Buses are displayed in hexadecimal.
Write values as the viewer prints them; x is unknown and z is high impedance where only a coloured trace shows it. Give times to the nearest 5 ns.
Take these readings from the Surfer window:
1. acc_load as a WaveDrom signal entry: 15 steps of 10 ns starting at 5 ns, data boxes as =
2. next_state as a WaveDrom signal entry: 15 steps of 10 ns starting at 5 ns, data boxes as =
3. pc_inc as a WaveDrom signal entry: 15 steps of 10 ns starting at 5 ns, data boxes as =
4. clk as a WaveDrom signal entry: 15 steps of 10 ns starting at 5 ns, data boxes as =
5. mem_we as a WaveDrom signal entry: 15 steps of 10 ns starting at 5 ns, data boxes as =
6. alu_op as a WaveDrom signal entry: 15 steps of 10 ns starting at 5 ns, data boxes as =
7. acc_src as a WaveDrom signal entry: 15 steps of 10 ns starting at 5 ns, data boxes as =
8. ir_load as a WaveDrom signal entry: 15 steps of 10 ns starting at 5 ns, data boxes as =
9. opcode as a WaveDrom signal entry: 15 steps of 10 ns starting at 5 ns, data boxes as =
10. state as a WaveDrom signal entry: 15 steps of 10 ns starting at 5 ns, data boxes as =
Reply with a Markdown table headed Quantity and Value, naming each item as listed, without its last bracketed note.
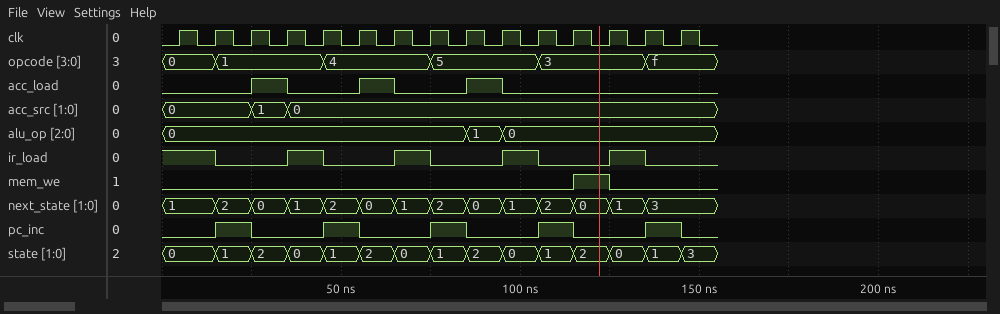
| Quantity | Value |
|---|---|
| acc_load as a WaveDrom signal entry: 15 steps of 10 ns starting at 5 ns, data boxes as = | {name: 'acc_load', wave: '0.10.10.10.....'} |
| next_state as a WaveDrom signal entry: 15 steps of 10 ns starting at 5 ns, data boxes as = | {name: 'next_state', wave: '==============.', data: '1 2 0 1 2 0 1 2 0 1 2 0 1 3'} |
| pc_inc as a WaveDrom signal entry: 15 steps of 10 ns starting at 5 ns, data boxes as = | {name: 'pc_inc', wave: '010.10.10.10.10'} |
| clk as a WaveDrom signal entry: 15 steps of 10 ns starting at 5 ns, data boxes as = | {name: 'clk', wave: 'p..............'} |
| mem_we as a WaveDrom signal entry: 15 steps of 10 ns starting at 5 ns, data boxes as = | {name: 'mem_we', wave: '0..........10..'} |
| alu_op as a WaveDrom signal entry: 15 steps of 10 ns starting at 5 ns, data boxes as = | {name: 'alu_op', wave: '=.......==.....', data: '0 1 0'} |
| acc_src as a WaveDrom signal entry: 15 steps of 10 ns starting at 5 ns, data boxes as = | {name: 'acc_src', wave: '=.==...........', data: '0 1 0'} |
| ir_load as a WaveDrom signal entry: 15 steps of 10 ns starting at 5 ns, data boxes as = | {name: 'ir_load', wave: '10.10.10.10.10.'} |
| opcode as a WaveDrom signal entry: 15 steps of 10 ns starting at 5 ns, data boxes as = | {name: 'opcode', wave: '==..=..=..=..=.', data: '0 1 4 5 3 f'} |
| state as a WaveDrom signal entry: 15 steps of 10 ns starting at 5 ns, data boxes as = | {name: 'state', wave: '===============', data: '0 1 2 0 1 2 0 1 2 0 1 2 0 1 3'} |
